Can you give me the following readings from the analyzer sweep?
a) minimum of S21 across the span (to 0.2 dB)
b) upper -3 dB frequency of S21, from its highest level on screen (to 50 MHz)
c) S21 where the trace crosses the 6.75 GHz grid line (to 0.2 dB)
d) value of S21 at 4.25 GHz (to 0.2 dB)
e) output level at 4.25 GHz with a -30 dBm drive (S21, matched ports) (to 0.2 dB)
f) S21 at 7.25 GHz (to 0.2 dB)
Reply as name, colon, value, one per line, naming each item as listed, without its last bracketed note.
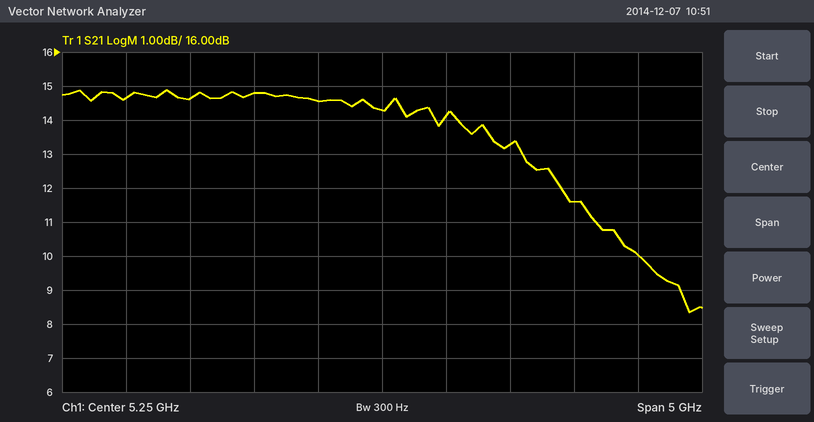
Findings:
minimum of S21 across the span: 8.4 dB
upper -3 dB frequency of S21, from its highest level on screen: 6.65 GHz
S21 where the trace crosses the 6.75 GHz grid line: 11.6 dB
value of S21 at 4.25 GHz: 14.8 dB
output level at 4.25 GHz with a -30 dBm drive (S21, matched ports): -15.2 dBm
S21 at 7.25 GHz: 10.0 dB
